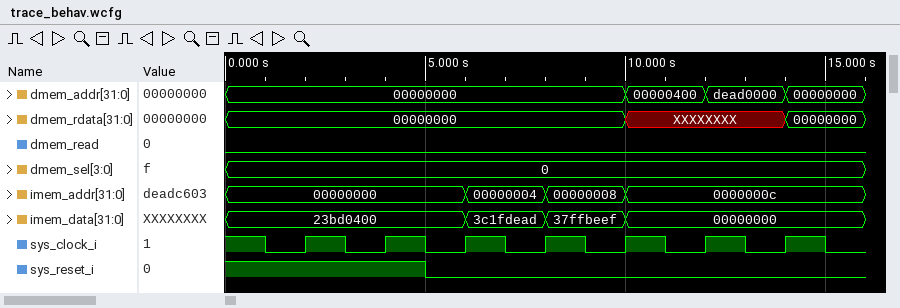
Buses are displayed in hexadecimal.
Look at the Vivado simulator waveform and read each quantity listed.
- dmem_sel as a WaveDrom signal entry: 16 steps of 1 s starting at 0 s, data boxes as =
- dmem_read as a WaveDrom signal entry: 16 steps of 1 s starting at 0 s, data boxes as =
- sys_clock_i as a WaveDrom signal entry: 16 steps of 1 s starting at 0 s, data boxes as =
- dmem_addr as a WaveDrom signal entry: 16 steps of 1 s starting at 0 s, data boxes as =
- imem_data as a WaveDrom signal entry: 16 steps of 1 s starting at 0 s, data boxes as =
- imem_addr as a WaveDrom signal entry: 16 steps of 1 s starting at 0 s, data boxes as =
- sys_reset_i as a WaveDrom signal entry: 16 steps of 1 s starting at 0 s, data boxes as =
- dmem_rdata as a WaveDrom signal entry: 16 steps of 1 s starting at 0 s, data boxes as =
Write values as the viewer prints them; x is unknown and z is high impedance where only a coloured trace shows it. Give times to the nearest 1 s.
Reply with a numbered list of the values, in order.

1. {name: 'dmem_sel', wave: '=...............', data: '0'}
2. {name: 'dmem_read', wave: '0...............'}
3. {name: 'sys_clock_i', wave: '1010101010101010'}
4. {name: 'dmem_addr', wave: '=.........=.=.=.', data: '00000000 00000400 dead0000 00000000'}
5. {name: 'imem_data', wave: '=.....=.=.=.....', data: '23bd0400 3c1fdead 37ffbeef 00000000'}
6. {name: 'imem_addr', wave: '=.....=.=.=.....', data: '00000000 00000004 00000008 0000000c'}
7. {name: 'sys_reset_i', wave: '1....0..........'}
8. {name: 'dmem_rdata', wave: '=.........x...=.', data: '00000000 00000000'}
